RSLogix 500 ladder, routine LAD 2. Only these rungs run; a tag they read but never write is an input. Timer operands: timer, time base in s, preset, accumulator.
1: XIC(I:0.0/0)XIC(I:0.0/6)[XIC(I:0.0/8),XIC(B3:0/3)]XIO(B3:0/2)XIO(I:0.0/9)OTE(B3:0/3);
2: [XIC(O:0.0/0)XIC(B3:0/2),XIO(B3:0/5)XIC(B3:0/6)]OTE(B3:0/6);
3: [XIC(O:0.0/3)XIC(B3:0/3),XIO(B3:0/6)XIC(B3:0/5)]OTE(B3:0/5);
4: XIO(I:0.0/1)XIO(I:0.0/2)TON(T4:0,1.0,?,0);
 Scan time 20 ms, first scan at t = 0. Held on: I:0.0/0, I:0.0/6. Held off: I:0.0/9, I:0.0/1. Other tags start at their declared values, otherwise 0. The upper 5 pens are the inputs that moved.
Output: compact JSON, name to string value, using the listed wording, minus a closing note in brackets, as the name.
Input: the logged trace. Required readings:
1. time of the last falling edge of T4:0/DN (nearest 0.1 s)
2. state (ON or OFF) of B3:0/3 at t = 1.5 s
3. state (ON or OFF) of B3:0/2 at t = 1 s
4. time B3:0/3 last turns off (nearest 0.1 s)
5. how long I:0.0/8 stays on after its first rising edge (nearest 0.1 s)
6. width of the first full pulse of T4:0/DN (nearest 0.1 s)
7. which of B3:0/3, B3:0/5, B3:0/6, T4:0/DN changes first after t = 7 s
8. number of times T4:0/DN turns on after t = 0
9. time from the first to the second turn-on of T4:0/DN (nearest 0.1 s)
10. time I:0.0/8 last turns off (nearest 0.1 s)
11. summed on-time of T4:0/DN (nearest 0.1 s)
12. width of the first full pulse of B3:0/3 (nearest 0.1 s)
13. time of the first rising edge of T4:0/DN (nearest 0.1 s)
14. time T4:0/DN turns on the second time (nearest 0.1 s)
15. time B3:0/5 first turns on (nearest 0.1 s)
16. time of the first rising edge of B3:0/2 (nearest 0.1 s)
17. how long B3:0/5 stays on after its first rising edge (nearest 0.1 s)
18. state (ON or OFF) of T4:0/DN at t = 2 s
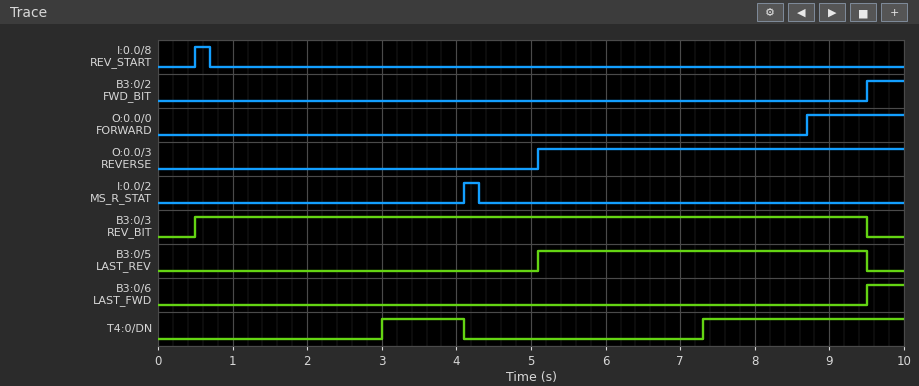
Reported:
{"time of the last falling edge of T4:0/DN": "4.1 s", "state (ON or OFF) of B3:0/3 at t = 1.5 s": "ON", "state (ON or OFF) of B3:0/2 at t = 1 s": "OFF", "time B3:0/3 last turns off": "9.5 s", "how long I:0.0/8 stays on after its first rising edge": "0.2 s", "width of the first full pulse of T4:0/DN": "1.1 s", "which of B3:0/3, B3:0/5, B3:0/6, T4:0/DN changes first after t = 7 s": "T4:0/DN", "number of times T4:0/DN turns on after t = 0": "2", "time from the first to the second turn-on of T4:0/DN": "4.3 s", "time I:0.0/8 last turns off": "0.7 s", "summed on-time of T4:0/DN": "3.8 s", "width of the first full pulse of B3:0/3": "9.0 s", "time of the first rising edge of T4:0/DN": "3.0 s", "time T4:0/DN turns on the second time": "7.3 s", "time B3:0/5 first turns on": "5.1 s", "time of the first rising edge of B3:0/2": "9.5 s", "how long B3:0/5 stays on after its first rising edge": "4.4 s", "state (ON or OFF) of T4:0/DN at t = 2 s": "OFF"}
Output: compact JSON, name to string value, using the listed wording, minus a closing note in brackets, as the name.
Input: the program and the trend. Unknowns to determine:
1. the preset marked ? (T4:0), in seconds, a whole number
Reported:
{"the preset marked ? (T4:0), in seconds, a whole number": "3 s"}
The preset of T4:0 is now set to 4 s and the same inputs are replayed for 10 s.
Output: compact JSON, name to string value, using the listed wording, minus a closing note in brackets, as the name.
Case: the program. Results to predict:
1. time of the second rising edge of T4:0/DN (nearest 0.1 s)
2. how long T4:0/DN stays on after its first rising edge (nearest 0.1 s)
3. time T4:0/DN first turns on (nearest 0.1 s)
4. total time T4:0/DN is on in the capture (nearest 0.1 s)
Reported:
{"time of the second rising edge of T4:0/DN": "8.3 s", "how long T4:0/DN stays on after its first rising edge": "0.1 s", "time T4:0/DN first turns on": "4.0 s", "total time T4:0/DN is on in the capture": "1.8 s"}
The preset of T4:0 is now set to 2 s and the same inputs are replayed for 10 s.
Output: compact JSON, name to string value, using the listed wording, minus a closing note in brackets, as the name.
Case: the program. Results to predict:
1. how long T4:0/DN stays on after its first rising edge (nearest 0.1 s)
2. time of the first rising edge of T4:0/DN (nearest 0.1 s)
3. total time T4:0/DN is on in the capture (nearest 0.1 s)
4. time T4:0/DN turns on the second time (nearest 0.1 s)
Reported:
{"how long T4:0/DN stays on after its first rising edge": "2.1 s", "time of the first rising edge of T4:0/DN": "2.0 s", "total time T4:0/DN is on in the capture": "5.8 s", "time T4:0/DN turns on the second time": "6.3 s"}
